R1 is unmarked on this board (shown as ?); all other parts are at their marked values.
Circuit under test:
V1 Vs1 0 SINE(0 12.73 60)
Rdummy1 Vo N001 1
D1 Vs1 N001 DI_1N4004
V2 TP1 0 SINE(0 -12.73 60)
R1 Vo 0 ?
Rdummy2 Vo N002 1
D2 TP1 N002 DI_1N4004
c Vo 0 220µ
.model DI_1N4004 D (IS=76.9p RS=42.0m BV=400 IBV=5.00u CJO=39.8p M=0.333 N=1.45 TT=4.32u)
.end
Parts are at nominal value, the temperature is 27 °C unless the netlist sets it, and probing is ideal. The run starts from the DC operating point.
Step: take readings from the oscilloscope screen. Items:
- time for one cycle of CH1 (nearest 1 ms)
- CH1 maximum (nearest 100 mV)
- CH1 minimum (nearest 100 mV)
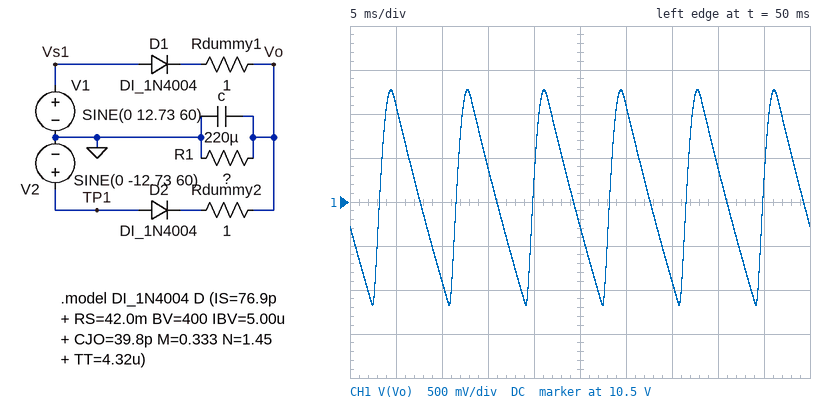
8 ms
11.8 V
9.3 V
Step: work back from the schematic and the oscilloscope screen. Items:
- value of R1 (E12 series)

120 Ω
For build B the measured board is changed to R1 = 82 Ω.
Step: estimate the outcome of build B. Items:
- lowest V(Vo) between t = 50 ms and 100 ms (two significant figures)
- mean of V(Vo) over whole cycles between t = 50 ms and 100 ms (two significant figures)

8.5 V
10 V
